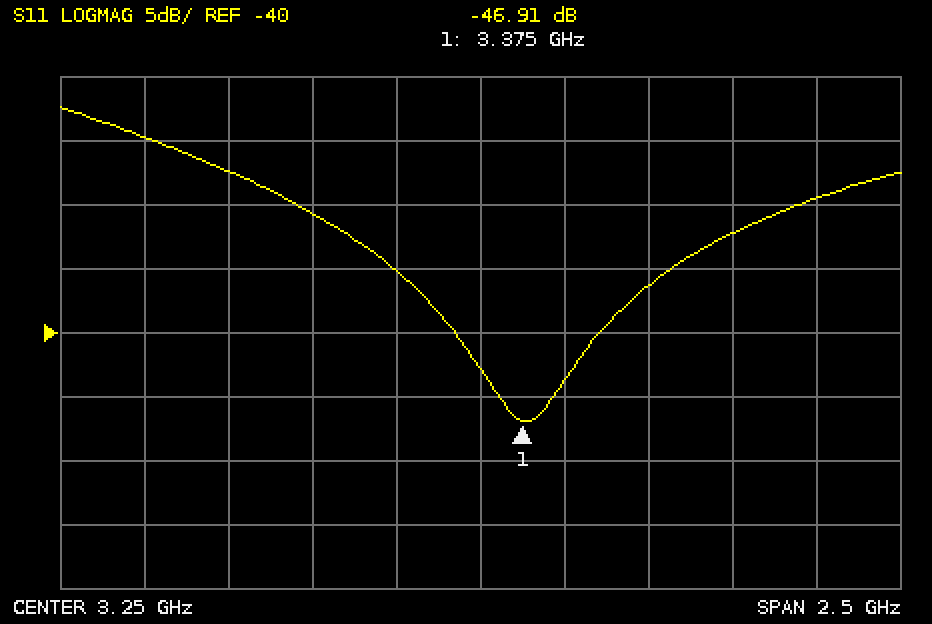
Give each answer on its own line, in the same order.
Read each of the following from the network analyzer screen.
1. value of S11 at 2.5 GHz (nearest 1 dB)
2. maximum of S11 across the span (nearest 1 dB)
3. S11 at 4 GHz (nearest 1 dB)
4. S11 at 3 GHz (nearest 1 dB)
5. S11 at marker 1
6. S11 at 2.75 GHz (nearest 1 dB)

-27 dB
-22 dB
-32 dB
-35 dB
-46.91 dB
-31 dB
